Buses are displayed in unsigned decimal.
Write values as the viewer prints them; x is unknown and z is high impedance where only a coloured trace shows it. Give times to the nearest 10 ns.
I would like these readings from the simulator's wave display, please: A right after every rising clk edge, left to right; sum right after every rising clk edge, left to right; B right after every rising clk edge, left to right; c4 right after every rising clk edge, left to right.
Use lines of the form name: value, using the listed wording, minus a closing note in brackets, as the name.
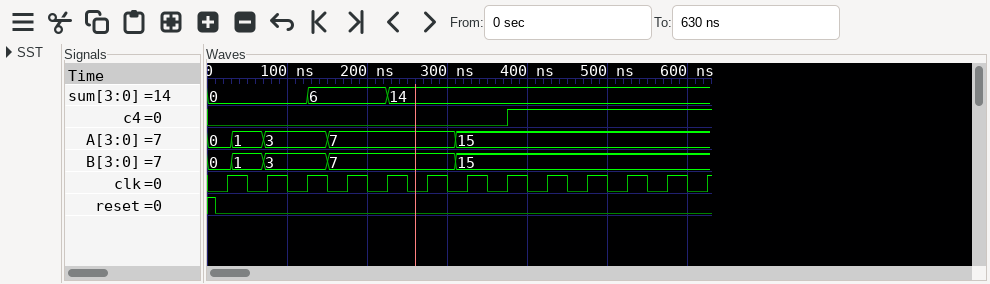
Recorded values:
A right after every rising clk edge, left to right: 0, 3, 3, 7, 7, 7, 15, 15, 15, 15, 15, 15, 15
sum right after every rising clk edge, left to right: 0, 0, 6, 6, 14, 14, 14, 14, 14, 14, 14, 14, 14
B right after every rising clk edge, left to right: 0, 3, 3, 7, 7, 7, 15, 15, 15, 15, 15, 15, 15
c4 right after every rising clk edge, left to right: 0 0 0 0 0 0 0 1 1 1 1 1 1
